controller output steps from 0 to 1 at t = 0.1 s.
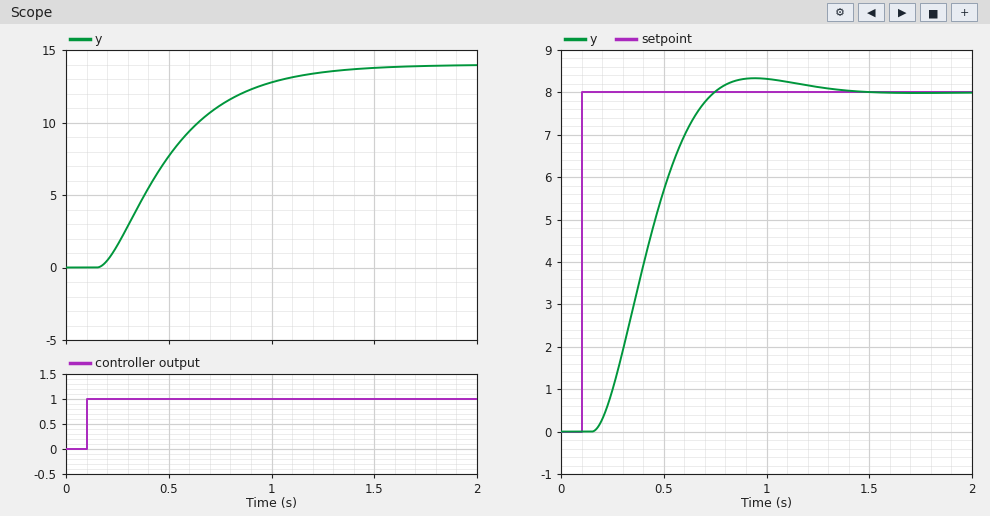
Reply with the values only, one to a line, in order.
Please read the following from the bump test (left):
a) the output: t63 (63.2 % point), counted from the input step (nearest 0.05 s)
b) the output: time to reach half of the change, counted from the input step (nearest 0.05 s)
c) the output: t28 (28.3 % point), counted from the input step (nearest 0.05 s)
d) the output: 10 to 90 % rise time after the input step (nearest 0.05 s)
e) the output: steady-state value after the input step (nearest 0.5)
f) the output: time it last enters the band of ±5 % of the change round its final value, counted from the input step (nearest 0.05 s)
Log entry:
0.45 s
0.35 s
0.25 s
0.70 s
14.0
1.05 s
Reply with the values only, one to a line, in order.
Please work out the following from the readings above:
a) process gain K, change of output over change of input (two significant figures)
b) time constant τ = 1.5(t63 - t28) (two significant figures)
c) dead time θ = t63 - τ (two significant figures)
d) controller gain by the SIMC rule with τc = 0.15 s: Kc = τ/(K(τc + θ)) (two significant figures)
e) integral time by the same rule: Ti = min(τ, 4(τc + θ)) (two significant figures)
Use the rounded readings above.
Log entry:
14
0.30 s
0.15 s
0.071
0.30 s
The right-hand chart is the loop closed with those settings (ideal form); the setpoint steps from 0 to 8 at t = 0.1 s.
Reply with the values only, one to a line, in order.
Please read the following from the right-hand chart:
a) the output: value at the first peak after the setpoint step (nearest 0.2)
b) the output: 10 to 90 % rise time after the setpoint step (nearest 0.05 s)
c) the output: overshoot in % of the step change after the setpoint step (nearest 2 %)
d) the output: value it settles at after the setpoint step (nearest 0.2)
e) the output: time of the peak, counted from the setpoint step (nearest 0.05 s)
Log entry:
8.4
0.40 s
4 %
8.0
0.85 s
